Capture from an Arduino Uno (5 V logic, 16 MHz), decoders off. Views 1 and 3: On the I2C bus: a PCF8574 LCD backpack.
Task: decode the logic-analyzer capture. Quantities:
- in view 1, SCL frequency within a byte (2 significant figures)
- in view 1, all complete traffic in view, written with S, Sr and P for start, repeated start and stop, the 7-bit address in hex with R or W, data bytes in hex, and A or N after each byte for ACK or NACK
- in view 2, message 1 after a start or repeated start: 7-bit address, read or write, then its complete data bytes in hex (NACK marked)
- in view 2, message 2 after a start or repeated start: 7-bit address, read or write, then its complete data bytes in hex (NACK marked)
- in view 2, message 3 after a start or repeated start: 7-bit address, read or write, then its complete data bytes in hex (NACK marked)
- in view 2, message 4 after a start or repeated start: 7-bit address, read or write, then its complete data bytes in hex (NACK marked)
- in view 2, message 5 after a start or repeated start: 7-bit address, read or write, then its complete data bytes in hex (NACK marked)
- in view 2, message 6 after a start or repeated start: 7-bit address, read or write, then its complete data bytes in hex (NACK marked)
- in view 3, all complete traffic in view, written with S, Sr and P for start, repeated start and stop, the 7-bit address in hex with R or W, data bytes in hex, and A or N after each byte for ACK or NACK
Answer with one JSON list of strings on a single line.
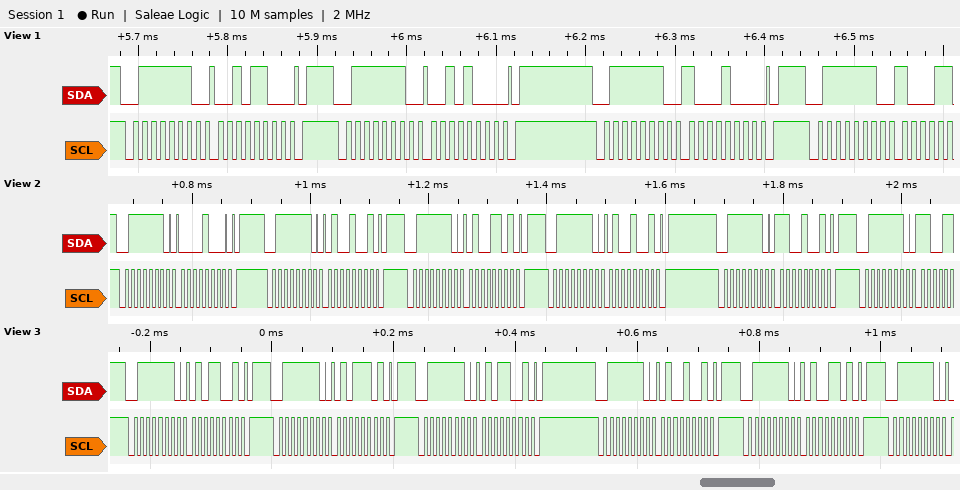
["100 kHz", "S 3FW A 2C A P S 3FW A 28 A P S 3FW A 88 A P S 3FW A", "0x3F write: 08", "0x3F write: 49", "0x3F write: 4D", "0x3F write: 49", "0x3F write: C9", "0x3F write", "S 3FW A 59 A P S 3FW A 5D A P S 3FW A 59 A P S 3FW A 49 A P S 3FW A 4D A P S 3FW A"]
